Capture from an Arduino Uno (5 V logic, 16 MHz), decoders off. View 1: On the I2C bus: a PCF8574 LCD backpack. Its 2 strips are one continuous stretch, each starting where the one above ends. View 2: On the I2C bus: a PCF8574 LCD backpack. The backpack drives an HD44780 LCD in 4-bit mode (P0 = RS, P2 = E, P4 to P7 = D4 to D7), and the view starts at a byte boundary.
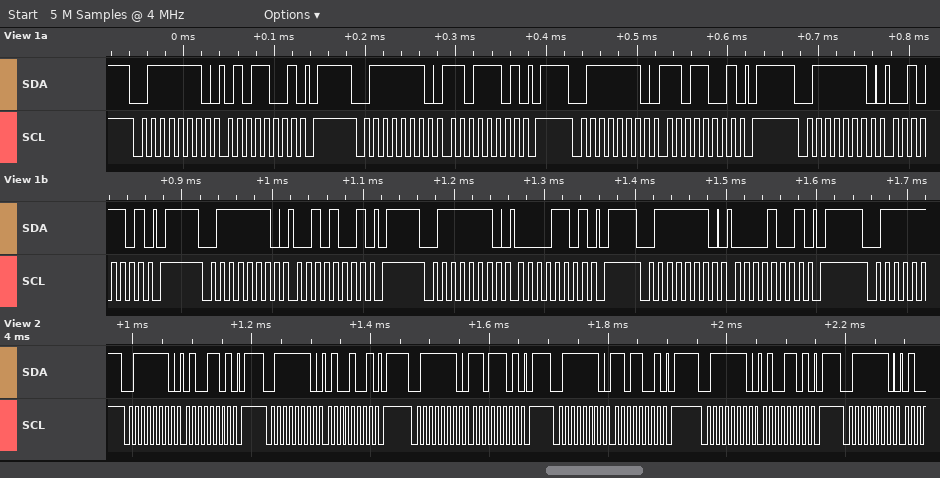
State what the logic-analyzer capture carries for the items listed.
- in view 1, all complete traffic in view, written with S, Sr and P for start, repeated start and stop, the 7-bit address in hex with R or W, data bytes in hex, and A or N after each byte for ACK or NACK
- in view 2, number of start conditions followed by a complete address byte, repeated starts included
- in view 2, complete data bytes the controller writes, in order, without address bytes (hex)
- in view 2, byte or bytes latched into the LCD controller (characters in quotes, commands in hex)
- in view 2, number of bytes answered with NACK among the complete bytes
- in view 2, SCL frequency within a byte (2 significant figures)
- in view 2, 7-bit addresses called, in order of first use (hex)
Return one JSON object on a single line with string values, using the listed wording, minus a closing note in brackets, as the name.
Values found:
{"in view 1, all complete traffic in view, written with S, Sr and P for start, repeated start and stop, the 7-bit address in hex with R or W, data bytes in hex, and A or N after each byte for ACK or NACK": "S 3FW A 59 A P S 3FW A DD A P S 3FW A D9 A P S 3FW A 2D A P S 3FW A 29 A P S 3FW A 0D A P S 3FW A 09 A P", "in view 2, number of start conditions followed by a complete address byte, repeated starts included": "6", "in view 2, complete data bytes the controller writes, in order, without address bytes": "4D 49 DD D9 4D", "in view 2, byte or bytes latched into the LCD controller": "'M'", "in view 2, number of bytes answered with NACK among the complete bytes": "0", "in view 2, SCL frequency within a byte": "100 kHz", "in view 2, 7-bit addresses called, in order of first use": "0x3F"}
